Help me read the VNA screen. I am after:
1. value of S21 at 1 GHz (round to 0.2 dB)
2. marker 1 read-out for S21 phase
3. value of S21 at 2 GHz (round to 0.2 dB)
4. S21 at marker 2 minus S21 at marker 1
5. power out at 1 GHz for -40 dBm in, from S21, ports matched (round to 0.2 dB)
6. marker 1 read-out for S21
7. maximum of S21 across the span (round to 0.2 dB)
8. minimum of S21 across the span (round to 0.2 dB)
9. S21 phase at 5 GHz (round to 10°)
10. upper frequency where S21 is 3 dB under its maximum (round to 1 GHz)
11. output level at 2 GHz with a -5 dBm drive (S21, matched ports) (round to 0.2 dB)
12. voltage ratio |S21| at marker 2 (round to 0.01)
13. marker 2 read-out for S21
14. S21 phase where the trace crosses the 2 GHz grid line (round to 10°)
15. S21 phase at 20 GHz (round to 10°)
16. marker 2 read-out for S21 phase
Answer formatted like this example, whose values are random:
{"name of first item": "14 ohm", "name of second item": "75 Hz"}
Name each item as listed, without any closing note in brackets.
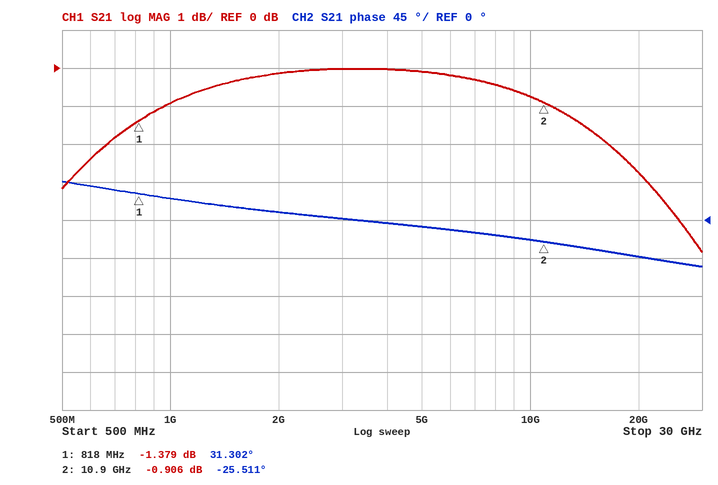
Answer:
{"value of S21 at 1 GHz": "-1.0 dB", "marker 1 read-out for S21 phase": "31.302°", "value of S21 at 2 GHz": "-0.2 dB", "S21 at marker 2 minus S21 at marker 1": "0.473 dB", "power out at 1 GHz for -40 dBm in, from S21, ports matched": "-41.0 dBm", "marker 1 read-out for S21": "-1.379 dB", "maximum of S21 across the span": "0.0 dB", "minimum of S21 across the span": "-4.8 dB", "S21 phase at 5 GHz": "-10°", "upper frequency where S21 is 3 dB under its maximum": "21 GHz", "output level at 2 GHz with a -5 dBm drive (S21, matched ports)": "-5.2 dBm", "voltage ratio |S21| at marker 2": "0.90", "marker 2 read-out for S21": "-0.906 dB", "S21 phase where the trace crosses the 2 GHz grid line": "10°", "S21 phase at 20 GHz": "-40°", "marker 2 read-out for S21 phase": "-25.511°"}
